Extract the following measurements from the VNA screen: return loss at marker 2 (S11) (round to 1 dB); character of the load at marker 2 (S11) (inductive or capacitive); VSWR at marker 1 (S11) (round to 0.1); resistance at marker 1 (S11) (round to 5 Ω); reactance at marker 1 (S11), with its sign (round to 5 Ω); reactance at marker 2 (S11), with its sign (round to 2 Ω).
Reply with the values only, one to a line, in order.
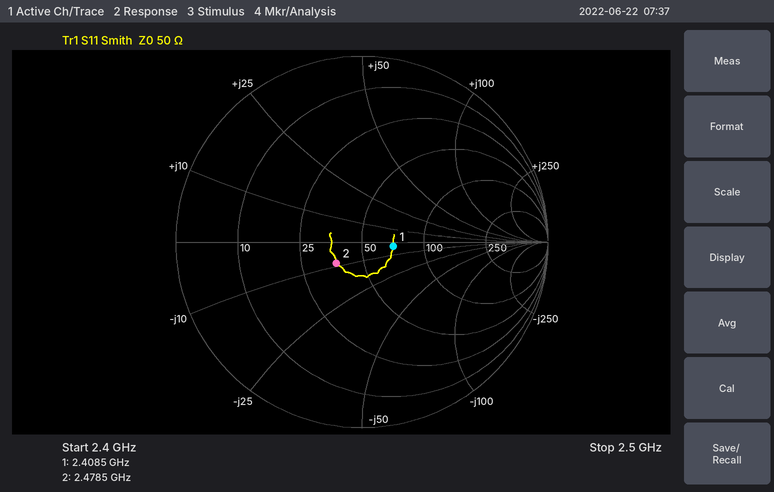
15 dB
capacitive
1.4
70 Ω
-5 Ω
-8 Ω
